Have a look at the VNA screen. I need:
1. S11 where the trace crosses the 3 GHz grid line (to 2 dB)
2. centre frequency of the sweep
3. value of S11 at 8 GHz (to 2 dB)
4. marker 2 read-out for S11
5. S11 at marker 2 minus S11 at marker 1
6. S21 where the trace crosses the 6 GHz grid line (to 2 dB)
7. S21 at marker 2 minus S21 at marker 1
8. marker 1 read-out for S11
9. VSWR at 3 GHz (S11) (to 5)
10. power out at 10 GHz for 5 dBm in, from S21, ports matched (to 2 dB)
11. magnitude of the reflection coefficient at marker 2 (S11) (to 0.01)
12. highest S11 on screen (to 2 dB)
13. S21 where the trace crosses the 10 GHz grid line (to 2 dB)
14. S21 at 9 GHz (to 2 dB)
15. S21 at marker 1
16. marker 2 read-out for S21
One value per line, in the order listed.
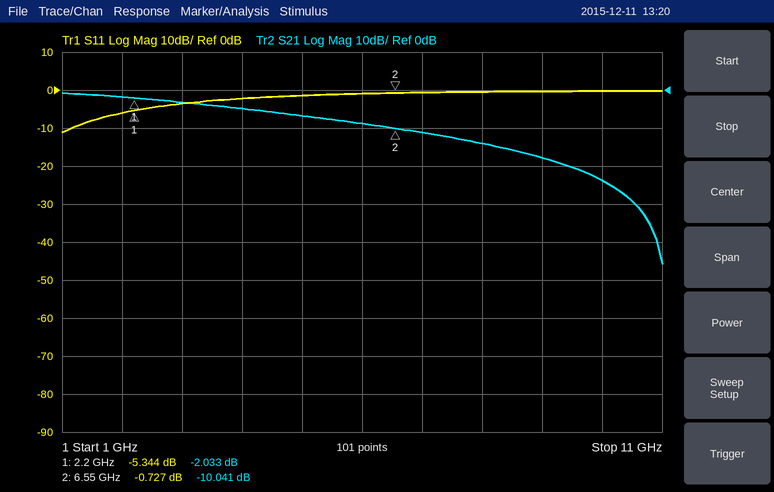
-4 dB
6 GHz
0 dB
-0.727 dB
4.617 dB
-8 dB
-8.008 dB
-5.344 dB
5
-18 dBm
0.92
0 dB
-24 dB
-18 dB
-2.033 dB
-10.041 dB
